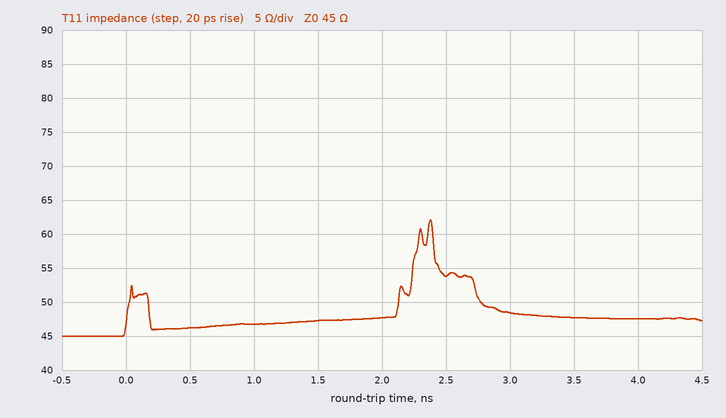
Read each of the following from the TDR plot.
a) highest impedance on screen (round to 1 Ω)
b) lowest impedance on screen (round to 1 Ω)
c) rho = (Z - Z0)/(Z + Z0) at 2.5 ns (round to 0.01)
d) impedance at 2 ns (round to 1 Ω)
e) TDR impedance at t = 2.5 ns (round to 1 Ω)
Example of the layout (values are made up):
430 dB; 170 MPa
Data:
62 Ω; 45 Ω; +0.09; 48 Ω; 54 Ω
